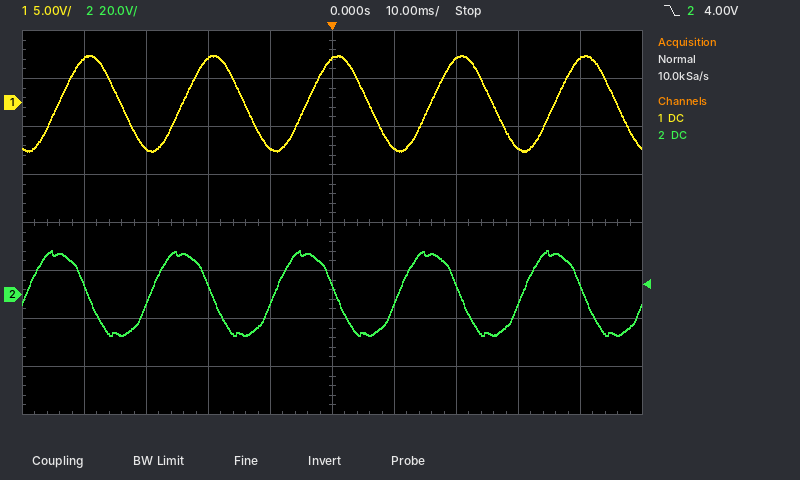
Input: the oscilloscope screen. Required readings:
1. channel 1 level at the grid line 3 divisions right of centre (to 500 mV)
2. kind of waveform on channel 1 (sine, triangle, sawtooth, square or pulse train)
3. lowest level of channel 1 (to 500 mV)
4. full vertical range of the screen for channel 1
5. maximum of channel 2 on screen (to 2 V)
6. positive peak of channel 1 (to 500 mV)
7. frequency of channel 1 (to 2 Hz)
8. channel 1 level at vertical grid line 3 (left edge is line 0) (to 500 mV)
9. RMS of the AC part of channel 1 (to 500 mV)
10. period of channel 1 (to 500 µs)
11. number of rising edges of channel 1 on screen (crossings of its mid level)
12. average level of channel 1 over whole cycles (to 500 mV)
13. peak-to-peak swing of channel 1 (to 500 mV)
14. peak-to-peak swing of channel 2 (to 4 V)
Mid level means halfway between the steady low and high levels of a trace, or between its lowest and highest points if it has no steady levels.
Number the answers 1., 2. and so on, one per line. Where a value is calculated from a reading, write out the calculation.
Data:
1. -4.5 V
2. sine
3. -5.0 V
4. 40 V
5. 18 V
6. 5.0 V
7. 1 / 20.0 ms ≈ 50 Hz
8. 4.5 V
9. 10.0 V / (2√2) ≈ 3.5 V
10. 20.0 ms
11. 5
12. (5.0 V + (-5.0 V)) / 2 ≈ 0.0 V
13. 5.0 V − (-5.0 V) = 10.0 V
14. 36 V
